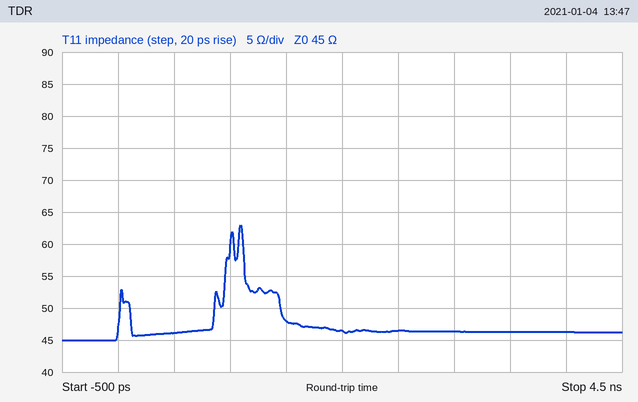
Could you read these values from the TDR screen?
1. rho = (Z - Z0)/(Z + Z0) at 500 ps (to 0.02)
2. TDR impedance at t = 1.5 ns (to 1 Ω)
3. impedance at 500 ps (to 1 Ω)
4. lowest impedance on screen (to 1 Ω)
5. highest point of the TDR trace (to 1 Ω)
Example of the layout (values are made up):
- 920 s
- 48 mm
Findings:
- +0.02
- 48 Ω
- 46 Ω
- 45 Ω
- 63 Ω
